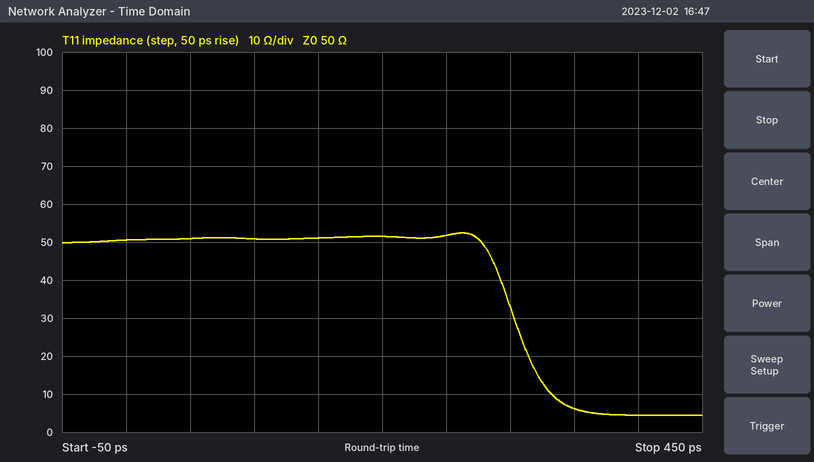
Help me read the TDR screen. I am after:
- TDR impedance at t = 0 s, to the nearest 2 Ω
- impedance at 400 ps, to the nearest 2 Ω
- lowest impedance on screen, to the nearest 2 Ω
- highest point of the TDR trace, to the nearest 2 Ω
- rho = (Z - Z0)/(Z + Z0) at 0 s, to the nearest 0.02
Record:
50 Ω
4 Ω
4 Ω
52 Ω
0.00
